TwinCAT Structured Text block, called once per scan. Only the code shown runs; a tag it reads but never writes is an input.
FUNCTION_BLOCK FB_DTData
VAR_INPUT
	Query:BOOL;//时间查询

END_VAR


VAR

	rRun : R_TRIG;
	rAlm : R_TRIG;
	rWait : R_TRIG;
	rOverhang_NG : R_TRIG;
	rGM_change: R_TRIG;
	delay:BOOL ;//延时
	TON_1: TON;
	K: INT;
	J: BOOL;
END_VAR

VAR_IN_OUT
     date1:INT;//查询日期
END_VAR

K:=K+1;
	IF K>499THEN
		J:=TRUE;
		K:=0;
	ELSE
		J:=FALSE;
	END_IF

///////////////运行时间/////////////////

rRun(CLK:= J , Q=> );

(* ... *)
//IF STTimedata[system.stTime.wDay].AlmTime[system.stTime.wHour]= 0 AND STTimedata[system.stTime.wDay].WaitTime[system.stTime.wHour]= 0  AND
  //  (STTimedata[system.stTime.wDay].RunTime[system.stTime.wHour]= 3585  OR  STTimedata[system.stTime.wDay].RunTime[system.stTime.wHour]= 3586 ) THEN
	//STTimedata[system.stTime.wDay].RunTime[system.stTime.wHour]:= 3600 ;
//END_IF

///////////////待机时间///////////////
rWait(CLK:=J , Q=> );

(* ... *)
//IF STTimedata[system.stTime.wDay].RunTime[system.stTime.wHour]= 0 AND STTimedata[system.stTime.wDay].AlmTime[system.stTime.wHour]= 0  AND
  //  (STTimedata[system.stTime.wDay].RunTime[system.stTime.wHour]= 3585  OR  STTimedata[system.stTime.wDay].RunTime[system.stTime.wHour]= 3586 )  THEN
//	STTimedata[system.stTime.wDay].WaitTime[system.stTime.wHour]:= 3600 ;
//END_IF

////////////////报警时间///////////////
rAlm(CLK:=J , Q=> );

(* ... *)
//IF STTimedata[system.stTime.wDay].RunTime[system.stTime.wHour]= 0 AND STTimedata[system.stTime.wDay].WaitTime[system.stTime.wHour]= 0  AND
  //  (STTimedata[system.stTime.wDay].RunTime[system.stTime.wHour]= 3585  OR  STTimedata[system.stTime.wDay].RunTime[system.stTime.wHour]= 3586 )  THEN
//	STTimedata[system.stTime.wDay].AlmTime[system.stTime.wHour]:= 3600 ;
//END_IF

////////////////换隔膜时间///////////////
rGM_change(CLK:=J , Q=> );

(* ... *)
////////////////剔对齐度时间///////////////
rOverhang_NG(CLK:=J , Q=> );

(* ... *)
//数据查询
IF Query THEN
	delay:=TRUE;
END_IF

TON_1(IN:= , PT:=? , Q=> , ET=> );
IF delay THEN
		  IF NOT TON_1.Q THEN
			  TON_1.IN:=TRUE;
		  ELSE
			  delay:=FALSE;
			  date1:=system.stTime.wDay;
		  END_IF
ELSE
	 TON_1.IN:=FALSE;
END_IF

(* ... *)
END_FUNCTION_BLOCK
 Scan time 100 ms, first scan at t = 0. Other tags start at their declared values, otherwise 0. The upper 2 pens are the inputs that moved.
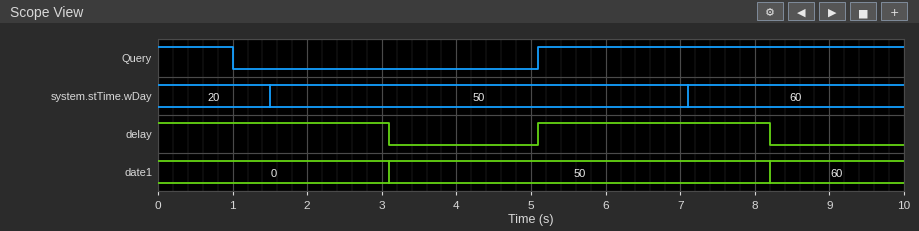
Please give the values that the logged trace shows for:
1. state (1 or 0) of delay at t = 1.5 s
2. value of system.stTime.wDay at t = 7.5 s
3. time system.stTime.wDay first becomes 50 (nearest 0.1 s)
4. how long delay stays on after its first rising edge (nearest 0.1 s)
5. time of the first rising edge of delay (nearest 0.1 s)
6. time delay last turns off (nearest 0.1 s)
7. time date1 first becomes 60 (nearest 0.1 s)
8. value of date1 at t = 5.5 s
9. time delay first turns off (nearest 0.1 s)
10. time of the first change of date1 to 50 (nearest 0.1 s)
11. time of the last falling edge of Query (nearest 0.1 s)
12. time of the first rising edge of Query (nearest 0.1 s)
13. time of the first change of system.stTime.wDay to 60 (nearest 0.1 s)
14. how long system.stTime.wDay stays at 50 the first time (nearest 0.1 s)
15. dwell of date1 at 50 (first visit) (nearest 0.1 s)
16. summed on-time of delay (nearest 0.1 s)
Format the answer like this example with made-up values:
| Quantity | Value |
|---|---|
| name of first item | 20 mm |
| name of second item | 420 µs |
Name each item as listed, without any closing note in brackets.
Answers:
| Quantity | Value |
|---|---|
| state (1 or 0) of delay at t = 1.5 s | 1 |
| value of system.stTime.wDay at t = 7.5 s | 60 |
| time system.stTime.wDay first becomes 50 | 1.5 s |
| how long delay stays on after its first rising edge | 3.1 s |
| time of the first rising edge of delay | 5.1 s |
| time delay last turns off | 8.2 s |
| time date1 first becomes 60 | 8.2 s |
| value of date1 at t = 5.5 s | 50 |
| time delay first turns off | 3.1 s |
| time of the first change of date1 to 50 | 3.1 s |
| time of the last falling edge of Query | 1.0 s |
| time of the first rising edge of Query | 5.1 s |
| time of the first change of system.stTime.wDay to 60 | 7.1 s |
| how long system.stTime.wDay stays at 50 the first time | 5.6 s |
| dwell of date1 at 50 (first visit) | 5.1 s |
| summed on-time of delay | 6.2 s |
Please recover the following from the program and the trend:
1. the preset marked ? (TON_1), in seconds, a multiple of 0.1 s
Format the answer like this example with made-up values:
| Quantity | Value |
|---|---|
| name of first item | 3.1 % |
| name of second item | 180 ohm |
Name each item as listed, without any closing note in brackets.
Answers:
| Quantity | Value |
|---|---|
| the preset marked ? (TON_1), in seconds, a multiple of 0.1 s | 3.0 s |
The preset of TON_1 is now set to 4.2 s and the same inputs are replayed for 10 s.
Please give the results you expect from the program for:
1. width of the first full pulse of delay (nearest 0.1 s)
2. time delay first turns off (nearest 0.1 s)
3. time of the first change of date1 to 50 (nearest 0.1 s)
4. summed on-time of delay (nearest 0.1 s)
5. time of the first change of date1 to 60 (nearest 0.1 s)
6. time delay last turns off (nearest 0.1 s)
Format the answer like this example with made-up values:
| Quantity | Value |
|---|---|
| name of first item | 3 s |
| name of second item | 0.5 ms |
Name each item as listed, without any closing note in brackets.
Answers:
| Quantity | Value |
|---|---|
| width of the first full pulse of delay | 4.3 s |
| time delay first turns off | 4.3 s |
| time of the first change of date1 to 50 | 4.3 s |
| summed on-time of delay | 8.6 s |
| time of the first change of date1 to 60 | 9.4 s |
| time delay last turns off | 9.4 s |
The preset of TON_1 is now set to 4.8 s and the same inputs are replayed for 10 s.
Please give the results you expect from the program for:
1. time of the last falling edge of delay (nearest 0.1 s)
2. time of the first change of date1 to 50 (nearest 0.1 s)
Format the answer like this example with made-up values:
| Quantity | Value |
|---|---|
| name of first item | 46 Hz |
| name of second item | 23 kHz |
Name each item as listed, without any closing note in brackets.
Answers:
| Quantity | Value |
|---|---|
| time of the last falling edge of delay | 4.9 s |
| time of the first change of date1 to 50 | 4.9 s |
